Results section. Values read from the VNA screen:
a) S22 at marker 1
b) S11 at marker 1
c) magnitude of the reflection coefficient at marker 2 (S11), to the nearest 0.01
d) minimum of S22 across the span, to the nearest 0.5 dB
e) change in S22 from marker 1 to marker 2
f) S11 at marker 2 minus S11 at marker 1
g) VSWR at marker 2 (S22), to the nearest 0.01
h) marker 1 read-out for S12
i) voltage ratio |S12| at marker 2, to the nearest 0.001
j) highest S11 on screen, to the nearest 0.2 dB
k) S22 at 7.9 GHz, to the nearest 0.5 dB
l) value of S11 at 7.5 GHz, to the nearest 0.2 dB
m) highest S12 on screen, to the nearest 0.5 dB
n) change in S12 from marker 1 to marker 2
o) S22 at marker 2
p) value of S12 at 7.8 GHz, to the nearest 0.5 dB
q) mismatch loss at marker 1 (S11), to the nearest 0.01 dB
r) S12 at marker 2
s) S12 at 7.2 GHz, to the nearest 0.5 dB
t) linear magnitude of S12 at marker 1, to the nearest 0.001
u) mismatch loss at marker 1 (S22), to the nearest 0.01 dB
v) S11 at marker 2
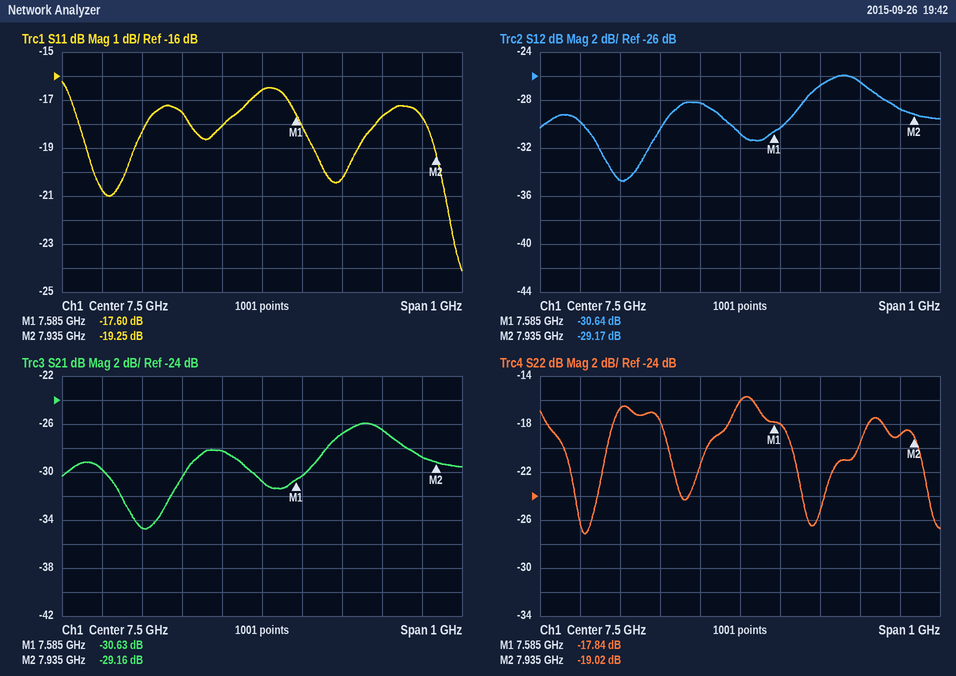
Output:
-17.84 dB
-17.60 dB
0.11
-27.0 dB
-1.18 dB
-1.65 dB
1.25
-30.64 dB
0.035
-16.2 dB
-19.0 dB
-16.6 dB
-26.0 dB
1.47 dB
-19.02 dB
-26.5 dB
0.08 dB
-29.17 dB
-34.5 dB
0.029
0.07 dB
-19.25 dB
